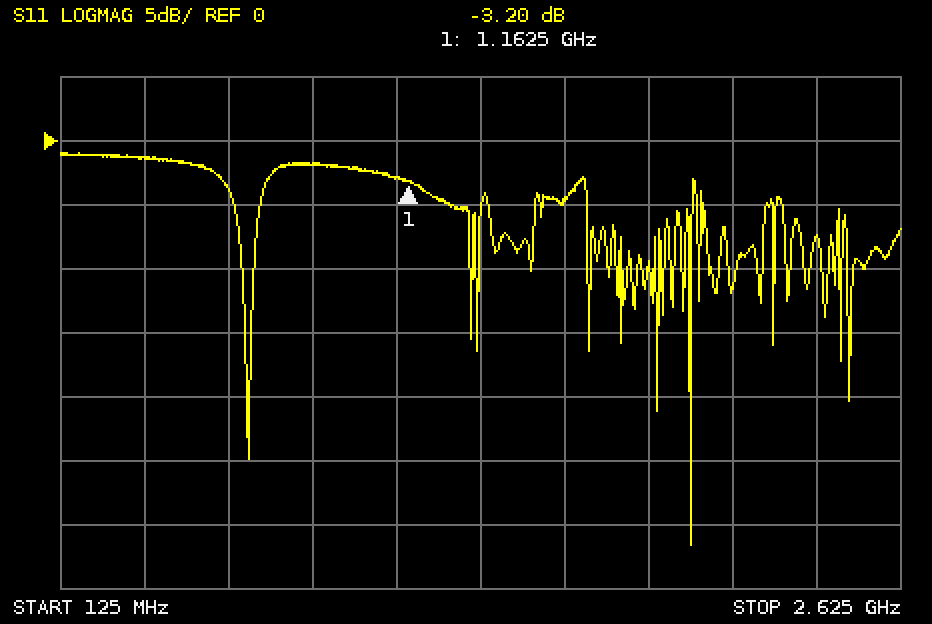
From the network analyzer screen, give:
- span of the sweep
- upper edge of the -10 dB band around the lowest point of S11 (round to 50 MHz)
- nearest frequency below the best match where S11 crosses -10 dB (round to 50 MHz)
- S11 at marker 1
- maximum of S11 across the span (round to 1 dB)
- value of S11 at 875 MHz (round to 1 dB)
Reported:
2.5 GHz
2.00 GHz
2.00 GHz
-3.20 dB
-1 dB
-2 dB
